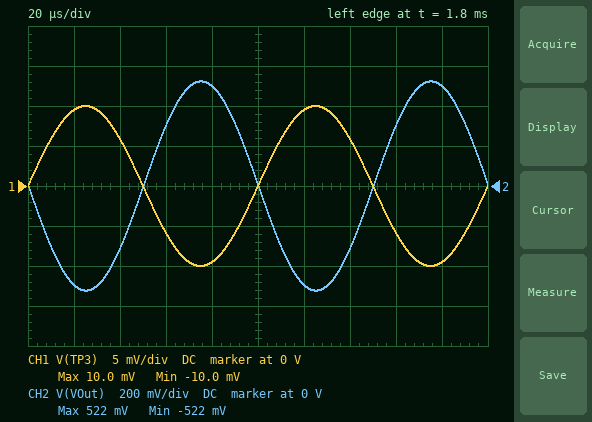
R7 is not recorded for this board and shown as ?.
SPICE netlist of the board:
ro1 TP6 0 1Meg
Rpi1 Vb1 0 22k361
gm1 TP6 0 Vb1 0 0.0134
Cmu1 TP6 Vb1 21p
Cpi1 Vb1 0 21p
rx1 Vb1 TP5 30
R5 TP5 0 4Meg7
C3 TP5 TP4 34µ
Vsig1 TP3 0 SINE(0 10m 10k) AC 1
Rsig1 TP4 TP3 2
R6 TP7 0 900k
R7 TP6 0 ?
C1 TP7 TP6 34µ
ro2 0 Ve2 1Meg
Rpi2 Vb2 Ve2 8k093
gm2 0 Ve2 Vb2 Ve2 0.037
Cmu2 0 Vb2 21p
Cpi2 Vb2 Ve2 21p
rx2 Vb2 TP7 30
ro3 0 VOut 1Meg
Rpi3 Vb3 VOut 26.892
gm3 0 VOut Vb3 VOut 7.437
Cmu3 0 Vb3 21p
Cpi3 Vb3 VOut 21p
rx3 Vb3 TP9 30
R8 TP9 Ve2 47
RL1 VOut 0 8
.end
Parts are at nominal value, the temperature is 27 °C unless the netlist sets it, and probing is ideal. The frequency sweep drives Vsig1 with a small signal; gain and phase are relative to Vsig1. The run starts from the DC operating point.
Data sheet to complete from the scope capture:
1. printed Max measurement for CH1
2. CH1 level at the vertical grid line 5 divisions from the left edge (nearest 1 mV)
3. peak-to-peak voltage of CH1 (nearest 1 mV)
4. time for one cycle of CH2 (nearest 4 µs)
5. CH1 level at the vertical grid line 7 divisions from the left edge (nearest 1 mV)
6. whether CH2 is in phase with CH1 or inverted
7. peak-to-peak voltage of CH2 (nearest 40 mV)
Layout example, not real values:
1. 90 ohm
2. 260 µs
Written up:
1. 10.0 mV
2. 0 V
3. 20 mV
4. 100 µs
5. 6 mV
6. inverted
7. 1.04 V
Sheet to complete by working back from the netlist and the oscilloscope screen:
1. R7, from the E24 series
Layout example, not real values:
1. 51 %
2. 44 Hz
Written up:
1. 4.3 kΩ
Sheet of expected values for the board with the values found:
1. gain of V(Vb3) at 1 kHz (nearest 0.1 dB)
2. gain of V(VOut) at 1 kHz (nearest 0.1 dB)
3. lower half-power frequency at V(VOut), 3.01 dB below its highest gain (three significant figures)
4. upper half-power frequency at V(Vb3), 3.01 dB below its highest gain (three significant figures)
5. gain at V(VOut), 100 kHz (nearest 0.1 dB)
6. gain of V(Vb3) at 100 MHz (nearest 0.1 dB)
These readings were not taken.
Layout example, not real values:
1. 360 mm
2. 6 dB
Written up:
1. 34.5 dB
2. 34.4 dB
3. 211 mHz
4. 731 kHz
5. 34.3 dB
6. -12.0 dB
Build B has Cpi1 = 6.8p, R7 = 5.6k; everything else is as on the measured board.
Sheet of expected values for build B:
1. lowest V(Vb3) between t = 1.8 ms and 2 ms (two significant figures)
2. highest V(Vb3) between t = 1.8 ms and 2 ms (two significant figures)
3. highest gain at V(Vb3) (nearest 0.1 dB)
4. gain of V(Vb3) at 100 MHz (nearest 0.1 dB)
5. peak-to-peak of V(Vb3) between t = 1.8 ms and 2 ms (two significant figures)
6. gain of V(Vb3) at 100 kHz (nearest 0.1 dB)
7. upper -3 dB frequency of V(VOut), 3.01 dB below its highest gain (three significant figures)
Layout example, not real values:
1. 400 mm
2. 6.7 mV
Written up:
1. -690 mV
2. 690 mV
3. 36.8 dB
4. -11.3 dB
5. 1.4 V
6. 36.6 dB
7. 565 kHz
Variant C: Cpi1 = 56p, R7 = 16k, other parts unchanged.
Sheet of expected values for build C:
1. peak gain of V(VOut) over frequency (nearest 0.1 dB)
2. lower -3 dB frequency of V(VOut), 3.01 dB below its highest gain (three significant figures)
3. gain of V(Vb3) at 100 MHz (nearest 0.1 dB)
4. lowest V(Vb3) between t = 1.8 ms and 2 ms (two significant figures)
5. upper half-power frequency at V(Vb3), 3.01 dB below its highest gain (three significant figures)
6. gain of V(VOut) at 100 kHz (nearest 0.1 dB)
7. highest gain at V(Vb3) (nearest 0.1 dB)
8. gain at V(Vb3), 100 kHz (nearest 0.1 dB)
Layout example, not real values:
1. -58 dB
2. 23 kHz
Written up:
1. 45.4 dB
2. 211 mHz
3. -14.3 dB
4. -1.9 V
5. 206 kHz
6. 44.5 dB
7. 45.5 dB
8. 44.6 dB
